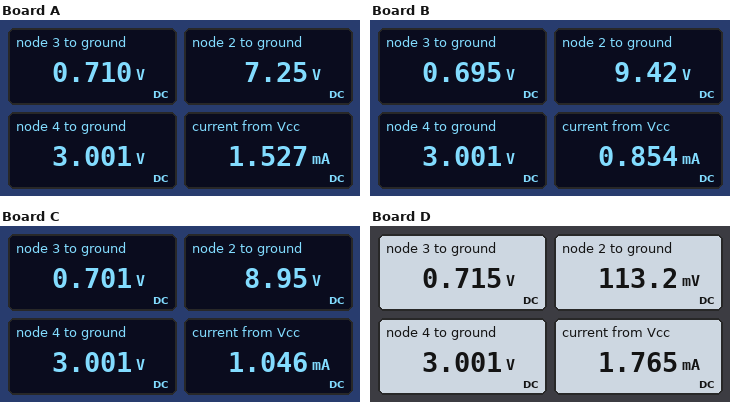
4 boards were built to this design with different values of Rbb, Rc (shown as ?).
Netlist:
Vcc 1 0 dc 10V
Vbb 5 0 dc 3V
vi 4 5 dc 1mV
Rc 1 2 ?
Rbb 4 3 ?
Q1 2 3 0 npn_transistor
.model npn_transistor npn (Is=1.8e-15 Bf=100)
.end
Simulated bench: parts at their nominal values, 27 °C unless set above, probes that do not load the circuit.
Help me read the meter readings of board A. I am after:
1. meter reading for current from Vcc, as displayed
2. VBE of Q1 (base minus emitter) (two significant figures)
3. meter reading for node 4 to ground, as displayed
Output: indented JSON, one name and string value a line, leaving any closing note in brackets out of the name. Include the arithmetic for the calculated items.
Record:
{
  "meter reading for current from Vcc, as displayed": "1.527 mA",
  "VBE of Q1 (base minus emitter)": "710 mV = 710 mV",
  "meter reading for node 4 to ground, as displayed": "3.001 V"
}
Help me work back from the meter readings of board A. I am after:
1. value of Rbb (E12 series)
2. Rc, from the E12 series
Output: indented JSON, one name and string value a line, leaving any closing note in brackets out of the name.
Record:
{
  "value of Rbb": "150 kΩ",
  "Rc, from the E12 series": "1.8 kΩ"
}
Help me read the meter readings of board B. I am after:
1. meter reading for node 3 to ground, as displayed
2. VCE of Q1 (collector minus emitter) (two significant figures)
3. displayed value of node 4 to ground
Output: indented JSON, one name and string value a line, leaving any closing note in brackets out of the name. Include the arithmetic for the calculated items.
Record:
{
  "meter reading for node 3 to ground, as displayed": "0.695 V",
  "VCE of Q1 (collector minus emitter)": "9.42 V = 9.4 V",
  "displayed value of node 4 to ground": "3.001 V"
}
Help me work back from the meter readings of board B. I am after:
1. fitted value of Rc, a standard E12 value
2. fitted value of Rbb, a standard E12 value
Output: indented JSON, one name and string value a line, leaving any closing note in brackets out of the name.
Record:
{
  "fitted value of Rc, a standard E12 value": "680 Ω",
  "fitted value of Rbb, a standard E12 value": "270 kΩ"
}
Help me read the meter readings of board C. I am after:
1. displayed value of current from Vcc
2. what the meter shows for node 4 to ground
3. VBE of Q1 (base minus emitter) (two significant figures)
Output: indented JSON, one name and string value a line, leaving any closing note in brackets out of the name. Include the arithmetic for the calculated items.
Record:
{
  "displayed value of current from Vcc": "1.046 mA",
  "what the meter shows for node 4 to ground": "3.001 V",
  "VBE of Q1 (base minus emitter)": "701 mV = 700 mV"
}
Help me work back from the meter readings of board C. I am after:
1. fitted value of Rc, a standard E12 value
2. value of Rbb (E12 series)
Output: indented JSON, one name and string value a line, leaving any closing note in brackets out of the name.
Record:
{
  "fitted value of Rc, a standard E12 value": "1 kΩ",
  "value of Rbb": "220 kΩ"
}
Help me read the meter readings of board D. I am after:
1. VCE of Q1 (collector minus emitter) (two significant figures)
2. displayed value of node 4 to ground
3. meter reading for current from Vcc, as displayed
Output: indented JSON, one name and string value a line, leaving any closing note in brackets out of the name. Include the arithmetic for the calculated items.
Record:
{
  "VCE of Q1 (collector minus emitter)": "113.2 mV = 110 mV",
  "displayed value of node 4 to ground": "3.001 V",
  "meter reading for current from Vcc, as displayed": "1.765 mA"
}
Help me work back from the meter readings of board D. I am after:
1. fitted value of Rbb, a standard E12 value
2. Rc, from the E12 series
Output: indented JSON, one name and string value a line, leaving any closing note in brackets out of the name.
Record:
{
  "fitted value of Rbb, a standard E12 value": "56 kΩ",
  "Rc, from the E12 series": "5.6 kΩ"
}
